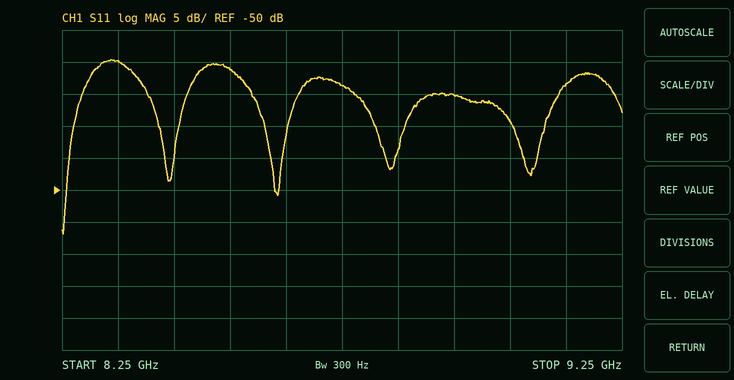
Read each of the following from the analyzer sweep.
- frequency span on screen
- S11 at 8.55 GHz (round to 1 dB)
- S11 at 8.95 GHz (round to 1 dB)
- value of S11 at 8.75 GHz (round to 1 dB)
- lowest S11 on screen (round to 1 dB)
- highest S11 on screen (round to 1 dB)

1 GHz
-31 dB
-35 dB
-34 dB
-57 dB
-30 dB
